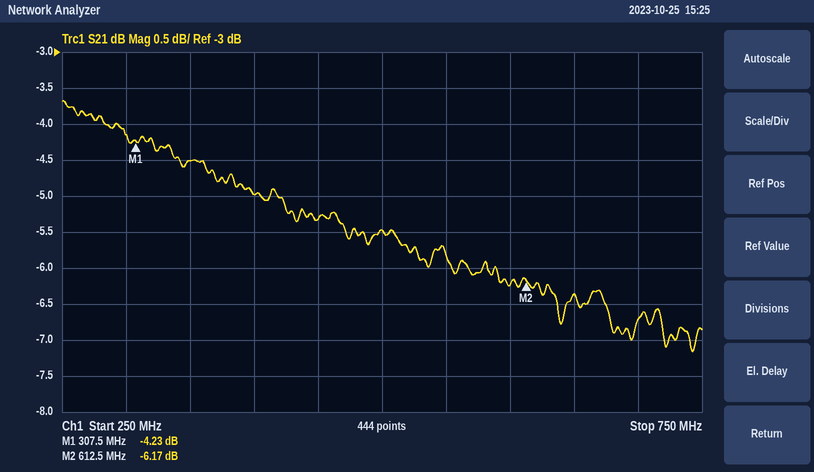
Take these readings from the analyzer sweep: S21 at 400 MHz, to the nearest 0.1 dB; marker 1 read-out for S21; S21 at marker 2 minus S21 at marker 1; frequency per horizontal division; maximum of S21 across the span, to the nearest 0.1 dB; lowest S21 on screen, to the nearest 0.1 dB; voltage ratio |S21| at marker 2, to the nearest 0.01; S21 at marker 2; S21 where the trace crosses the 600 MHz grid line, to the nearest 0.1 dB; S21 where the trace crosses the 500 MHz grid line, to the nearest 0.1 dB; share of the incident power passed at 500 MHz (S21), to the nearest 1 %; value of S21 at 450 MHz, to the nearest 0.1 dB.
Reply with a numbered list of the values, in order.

1. -5.0 dB
2. -4.23 dB
3. -1.94 dB
4. 50 MHz
5. -3.7 dB
6. -7.2 dB
7. 0.49
8. -6.17 dB
9. -6.2 dB
10. -5.5 dB
11. 28 %
12. -5.3 dB
